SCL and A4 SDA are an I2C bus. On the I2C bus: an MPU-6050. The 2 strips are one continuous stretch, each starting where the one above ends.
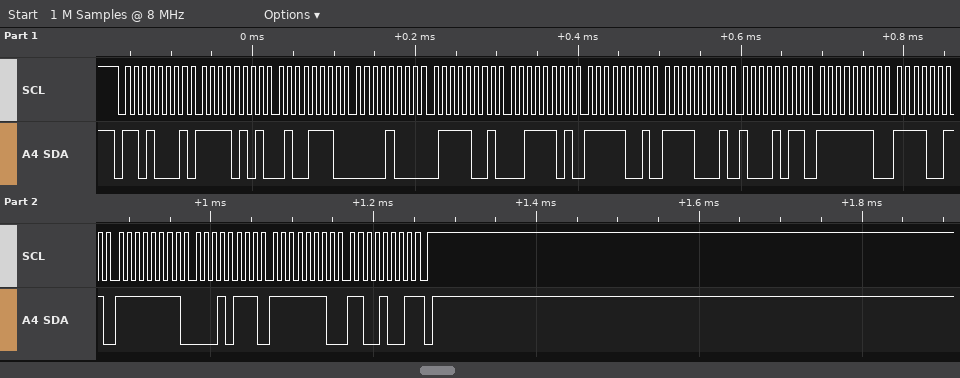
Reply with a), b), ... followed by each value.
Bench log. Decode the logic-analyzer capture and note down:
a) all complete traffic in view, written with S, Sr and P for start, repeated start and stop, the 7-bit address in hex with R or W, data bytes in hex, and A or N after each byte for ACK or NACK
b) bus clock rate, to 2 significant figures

a) S 68R A F5 A 4E A 08 A 79 A 3D A F9 A F1 A 8B A FE A F3 A FF A 17 A FE A C9 N P
b) 100 kHz
